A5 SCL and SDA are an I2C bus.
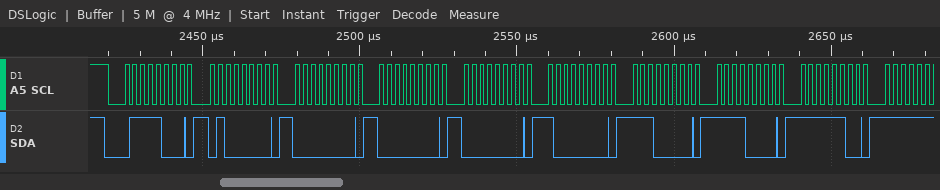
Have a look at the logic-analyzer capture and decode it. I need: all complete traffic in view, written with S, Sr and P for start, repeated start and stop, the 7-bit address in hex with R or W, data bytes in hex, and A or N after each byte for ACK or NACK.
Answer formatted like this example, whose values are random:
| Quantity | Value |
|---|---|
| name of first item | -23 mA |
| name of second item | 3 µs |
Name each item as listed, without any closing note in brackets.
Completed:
| Quantity | Value |
|---|---|
| all complete traffic in view, written with S, Sr and P for start, repeated start and stop, the 7-bit address in hex with R or W, data bytes in hex, and A or N after each byte for ACK or NACK | S 3CW A 40 A 00 A 00 A 00 A 80 A E0 A F0 A FC A |
